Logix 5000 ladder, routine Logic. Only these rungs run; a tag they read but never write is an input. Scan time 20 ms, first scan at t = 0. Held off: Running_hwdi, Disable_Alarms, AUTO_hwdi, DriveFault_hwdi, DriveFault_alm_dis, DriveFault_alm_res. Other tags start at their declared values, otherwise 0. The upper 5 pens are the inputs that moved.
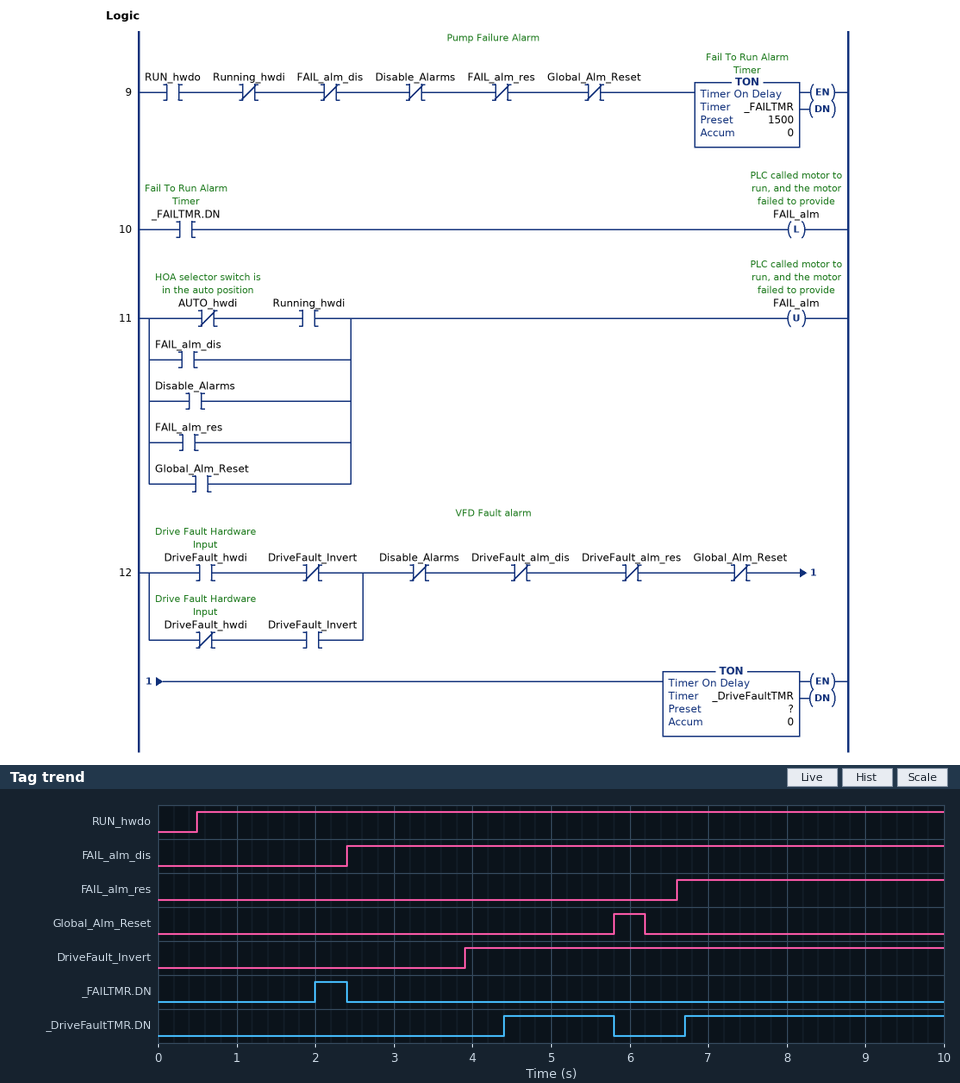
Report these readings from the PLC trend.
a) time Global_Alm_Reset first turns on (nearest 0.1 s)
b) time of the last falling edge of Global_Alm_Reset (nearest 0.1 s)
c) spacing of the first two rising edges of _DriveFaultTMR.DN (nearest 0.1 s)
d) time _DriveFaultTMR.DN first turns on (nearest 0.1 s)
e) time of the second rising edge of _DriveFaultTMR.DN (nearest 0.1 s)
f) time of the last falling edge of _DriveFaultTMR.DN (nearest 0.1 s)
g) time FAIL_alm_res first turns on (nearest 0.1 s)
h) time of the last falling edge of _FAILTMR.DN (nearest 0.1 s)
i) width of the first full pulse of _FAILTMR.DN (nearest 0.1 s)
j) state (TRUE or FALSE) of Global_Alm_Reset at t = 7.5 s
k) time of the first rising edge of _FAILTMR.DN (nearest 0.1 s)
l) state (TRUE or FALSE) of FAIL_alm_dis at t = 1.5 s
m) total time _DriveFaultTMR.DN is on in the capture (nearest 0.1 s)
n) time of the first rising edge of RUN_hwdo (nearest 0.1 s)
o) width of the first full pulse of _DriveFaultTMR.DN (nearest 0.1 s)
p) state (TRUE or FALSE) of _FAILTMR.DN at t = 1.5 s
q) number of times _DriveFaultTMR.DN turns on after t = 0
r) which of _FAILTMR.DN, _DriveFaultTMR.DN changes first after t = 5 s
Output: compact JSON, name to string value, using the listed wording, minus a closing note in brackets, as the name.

{"time Global_Alm_Reset first turns on": "5.8 s", "time of the last falling edge of Global_Alm_Reset": "6.2 s", "spacing of the first two rising edges of _DriveFaultTMR.DN": "2.3 s", "time _DriveFaultTMR.DN first turns on": "4.4 s", "time of the second rising edge of _DriveFaultTMR.DN": "6.7 s", "time of the last falling edge of _DriveFaultTMR.DN": "5.8 s", "time FAIL_alm_res first turns on": "6.6 s", "time of the last falling edge of _FAILTMR.DN": "2.4 s", "width of the first full pulse of _FAILTMR.DN": "0.4 s", "state (TRUE or FALSE) of Global_Alm_Reset at t = 7.5 s": "FALSE", "time of the first rising edge of _FAILTMR.DN": "2.0 s", "state (TRUE or FALSE) of FAIL_alm_dis at t = 1.5 s": "FALSE", "total time _DriveFaultTMR.DN is on in the capture": "4.7 s", "time of the first rising edge of RUN_hwdo": "0.5 s", "width of the first full pulse of _DriveFaultTMR.DN": "1.4 s", "state (TRUE or FALSE) of _FAILTMR.DN at t = 1.5 s": "FALSE", "number of times _DriveFaultTMR.DN turns on after t = 0": "2", "which of _FAILTMR.DN, _DriveFaultTMR.DN changes first after t = 5 s": "_DriveFaultTMR.DN"}
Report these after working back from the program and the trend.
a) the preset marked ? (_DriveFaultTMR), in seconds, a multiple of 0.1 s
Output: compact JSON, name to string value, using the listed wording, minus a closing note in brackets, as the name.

{"the preset marked ? (_DriveFaultTMR), in seconds, a multiple of 0.1 s": "0.5 s"}
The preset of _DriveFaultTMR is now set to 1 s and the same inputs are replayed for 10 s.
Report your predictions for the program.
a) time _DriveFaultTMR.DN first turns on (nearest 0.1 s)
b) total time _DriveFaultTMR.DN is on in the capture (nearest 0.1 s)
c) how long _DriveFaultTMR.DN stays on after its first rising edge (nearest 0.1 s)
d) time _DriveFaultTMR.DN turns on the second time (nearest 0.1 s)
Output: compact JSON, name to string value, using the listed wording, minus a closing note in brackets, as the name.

{"time _DriveFaultTMR.DN first turns on": "4.9 s", "total time _DriveFaultTMR.DN is on in the capture": "3.7 s", "how long _DriveFaultTMR.DN stays on after its first rising edge": "0.9 s", "time _DriveFaultTMR.DN turns on the second time": "7.2 s"}
